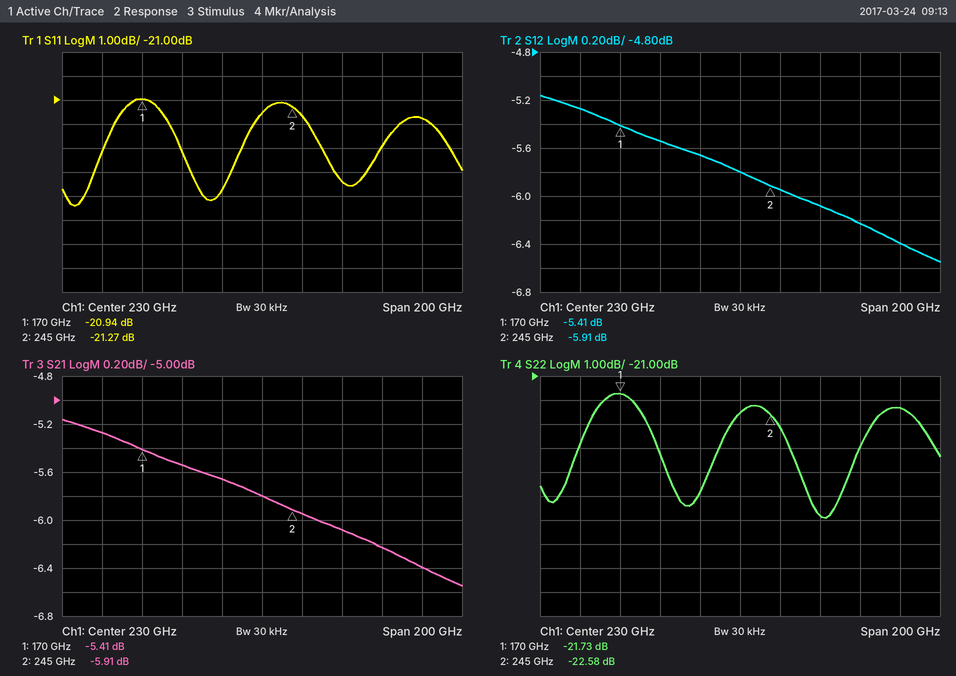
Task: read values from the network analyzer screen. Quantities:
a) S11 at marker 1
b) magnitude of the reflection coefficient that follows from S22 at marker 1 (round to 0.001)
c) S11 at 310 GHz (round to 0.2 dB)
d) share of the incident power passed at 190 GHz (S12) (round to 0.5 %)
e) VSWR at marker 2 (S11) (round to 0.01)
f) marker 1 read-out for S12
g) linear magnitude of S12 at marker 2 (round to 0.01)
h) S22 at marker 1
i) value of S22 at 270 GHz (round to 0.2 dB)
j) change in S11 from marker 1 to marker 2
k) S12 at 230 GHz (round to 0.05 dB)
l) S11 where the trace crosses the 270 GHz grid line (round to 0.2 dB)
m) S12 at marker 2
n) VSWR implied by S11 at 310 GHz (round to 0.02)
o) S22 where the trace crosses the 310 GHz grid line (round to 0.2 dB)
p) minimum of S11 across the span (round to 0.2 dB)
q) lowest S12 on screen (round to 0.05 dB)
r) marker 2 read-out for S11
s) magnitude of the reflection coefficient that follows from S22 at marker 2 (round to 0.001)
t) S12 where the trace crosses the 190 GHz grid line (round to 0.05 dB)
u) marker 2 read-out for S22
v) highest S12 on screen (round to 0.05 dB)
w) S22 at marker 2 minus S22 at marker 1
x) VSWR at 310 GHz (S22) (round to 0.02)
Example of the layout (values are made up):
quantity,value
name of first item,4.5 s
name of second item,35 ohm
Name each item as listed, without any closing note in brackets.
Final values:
quantity,value
S11 at marker 1,-20.94 dB
magnitude of the reflection coefficient that follows from S22 at marker 1,0.082
S11 at 310 GHz,-21.8 dB
share of the incident power passed at 190 GHz (S12),28.0 %
VSWR at marker 2 (S11),1.19
marker 1 read-out for S12,-5.41 dB
linear magnitude of S12 at marker 2,0.51
S22 at marker 1,-21.73 dB
value of S22 at 270 GHz,-26.8 dB
change in S11 from marker 1 to marker 2,-0.33 dB
S12 at 230 GHz,-5.80 dB
S11 where the trace crosses the 270 GHz grid line,-24.4 dB
S12 at marker 2,-5.91 dB
VSWR implied by S11 at 310 GHz,1.18
S22 where the trace crosses the 310 GHz grid line,-22.4 dB
minimum of S11 across the span,-25.4 dB
lowest S12 on screen,-6.55 dB
marker 2 read-out for S11,-21.27 dB
magnitude of the reflection coefficient that follows from S22 at marker 2,0.074
S12 where the trace crosses the 190 GHz grid line,-5.55 dB
marker 2 read-out for S22,-22.58 dB
highest S12 on screen,-5.15 dB
S22 at marker 2 minus S22 at marker 1,-0.85 dB
VSWR at 310 GHz (S22),1.16
